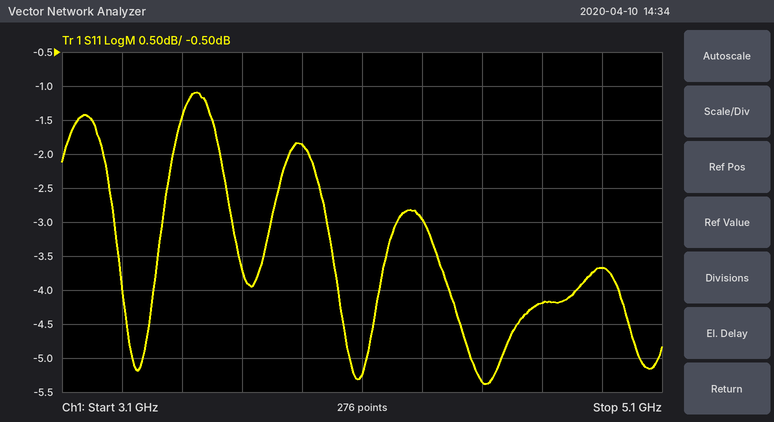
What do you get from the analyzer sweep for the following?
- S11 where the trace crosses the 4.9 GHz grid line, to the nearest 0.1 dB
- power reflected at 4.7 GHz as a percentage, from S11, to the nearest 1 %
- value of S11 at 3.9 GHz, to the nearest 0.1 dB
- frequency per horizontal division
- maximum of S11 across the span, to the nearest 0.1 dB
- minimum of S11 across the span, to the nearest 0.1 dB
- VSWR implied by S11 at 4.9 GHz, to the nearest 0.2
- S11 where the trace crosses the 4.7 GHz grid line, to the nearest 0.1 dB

-3.7 dB
38 %
-1.9 dB
200 MHz
-1.1 dB
-5.4 dB
4.8
-4.2 dB
